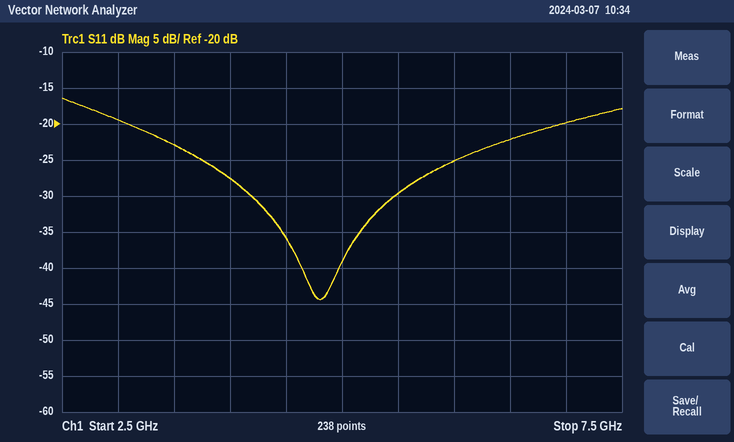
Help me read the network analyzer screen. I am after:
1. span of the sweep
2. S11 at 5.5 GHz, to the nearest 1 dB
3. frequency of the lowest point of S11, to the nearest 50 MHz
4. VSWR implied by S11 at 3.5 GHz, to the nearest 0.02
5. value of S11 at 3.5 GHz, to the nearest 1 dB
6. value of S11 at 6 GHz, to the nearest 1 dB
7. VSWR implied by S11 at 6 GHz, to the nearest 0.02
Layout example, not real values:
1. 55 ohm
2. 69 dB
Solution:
1. 5 GHz
2. -30 dB
3. 4.80 GHz
4. 1.16
5. -23 dB
6. -25 dB
7. 1.12
